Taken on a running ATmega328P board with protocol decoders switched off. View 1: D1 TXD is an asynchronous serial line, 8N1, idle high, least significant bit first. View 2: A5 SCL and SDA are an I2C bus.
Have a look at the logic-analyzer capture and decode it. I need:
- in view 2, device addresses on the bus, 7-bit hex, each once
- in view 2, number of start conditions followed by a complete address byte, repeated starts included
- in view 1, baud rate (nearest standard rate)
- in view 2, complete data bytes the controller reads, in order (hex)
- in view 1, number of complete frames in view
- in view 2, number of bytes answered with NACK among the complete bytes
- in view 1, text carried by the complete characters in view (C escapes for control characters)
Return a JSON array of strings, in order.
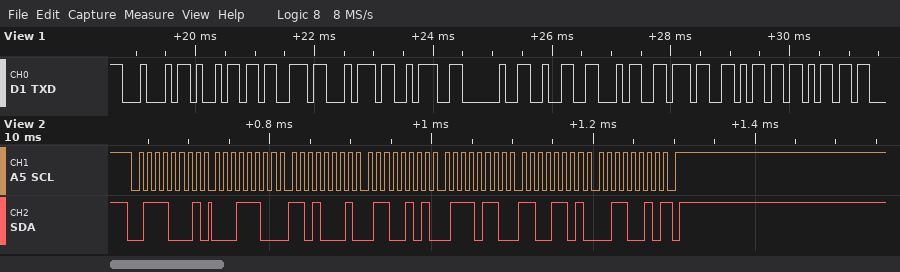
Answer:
["0x38", "1", "9600 baud", "1C D1 65 76 CD 32", "11", "1", "\"Dist: 247mm\""]
